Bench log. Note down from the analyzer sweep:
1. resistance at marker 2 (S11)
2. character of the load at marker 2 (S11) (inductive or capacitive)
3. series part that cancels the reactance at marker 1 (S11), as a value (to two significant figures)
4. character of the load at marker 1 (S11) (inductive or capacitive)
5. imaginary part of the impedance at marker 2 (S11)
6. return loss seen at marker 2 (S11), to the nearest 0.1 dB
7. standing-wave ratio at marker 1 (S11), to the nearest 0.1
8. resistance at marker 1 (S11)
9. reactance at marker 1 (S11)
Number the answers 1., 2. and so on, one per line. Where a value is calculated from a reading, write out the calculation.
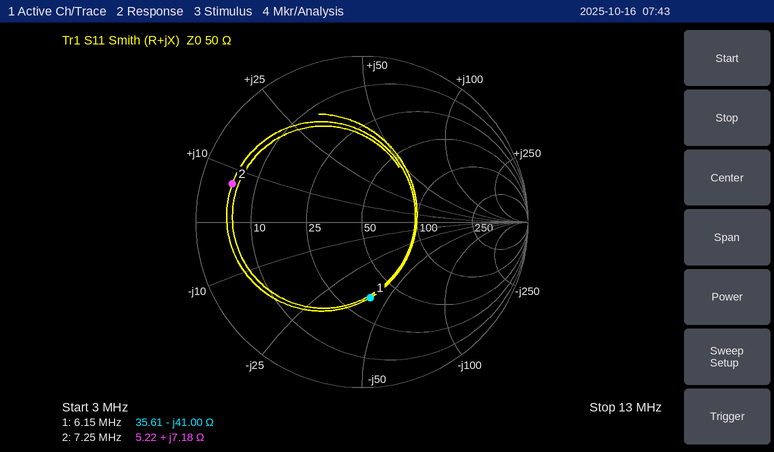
1. 5.22 Ω
2. inductive
3. L = 41 Ω/(2π × 6.15 MHz) ≈ 1.1 µH
4. capacitive
5. +7.18 Ω
6. 1.8 dB
7. 2.7
8. 35.61 Ω
9. -41.00 Ω
